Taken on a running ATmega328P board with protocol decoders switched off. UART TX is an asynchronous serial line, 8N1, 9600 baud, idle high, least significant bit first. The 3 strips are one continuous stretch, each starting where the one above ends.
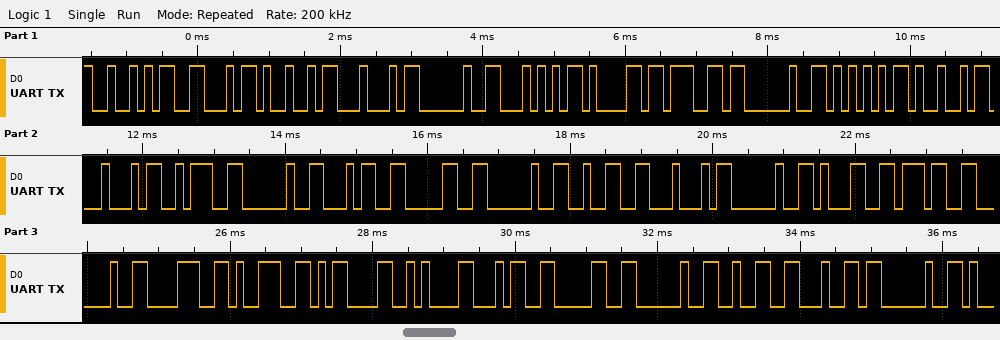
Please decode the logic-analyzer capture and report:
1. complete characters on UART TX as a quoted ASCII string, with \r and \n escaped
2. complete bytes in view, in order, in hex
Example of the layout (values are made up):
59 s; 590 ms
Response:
"RFID Tag UID: 40 2D 17 89\r\n40 2d "; 52 46 49 44 20 54 61 67 20 55 49 44 3A 20 34 30 20 32 44 20 31 37 20 38 39 0D 0A 34 30 20 32 64 20
